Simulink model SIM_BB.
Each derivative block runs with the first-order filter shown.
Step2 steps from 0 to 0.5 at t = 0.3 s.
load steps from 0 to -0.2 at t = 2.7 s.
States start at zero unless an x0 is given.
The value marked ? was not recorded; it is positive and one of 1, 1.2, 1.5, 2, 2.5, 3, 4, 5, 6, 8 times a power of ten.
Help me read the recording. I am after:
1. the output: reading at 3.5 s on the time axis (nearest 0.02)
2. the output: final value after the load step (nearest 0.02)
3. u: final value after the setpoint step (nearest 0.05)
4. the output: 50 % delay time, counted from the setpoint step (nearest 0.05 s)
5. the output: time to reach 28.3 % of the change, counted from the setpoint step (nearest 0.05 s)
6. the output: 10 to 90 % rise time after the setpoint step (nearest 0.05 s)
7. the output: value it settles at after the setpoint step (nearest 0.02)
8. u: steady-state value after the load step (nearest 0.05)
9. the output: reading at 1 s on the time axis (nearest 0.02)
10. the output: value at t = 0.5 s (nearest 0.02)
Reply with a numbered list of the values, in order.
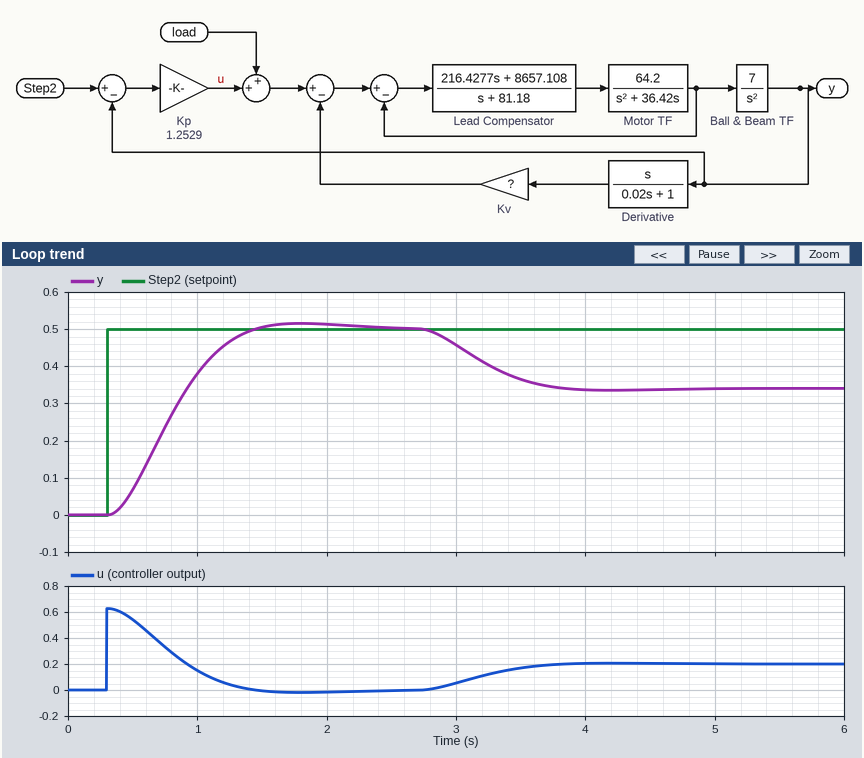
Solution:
1. 0.36
2. 0.34
3. 0.00
4. 0.45 s
5. 0.30 s
6. 0.70 s
7. 0.50
8. 0.20
9. 0.38
10. 0.06
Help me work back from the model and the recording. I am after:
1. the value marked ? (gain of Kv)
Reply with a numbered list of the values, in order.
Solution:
1. 0.6
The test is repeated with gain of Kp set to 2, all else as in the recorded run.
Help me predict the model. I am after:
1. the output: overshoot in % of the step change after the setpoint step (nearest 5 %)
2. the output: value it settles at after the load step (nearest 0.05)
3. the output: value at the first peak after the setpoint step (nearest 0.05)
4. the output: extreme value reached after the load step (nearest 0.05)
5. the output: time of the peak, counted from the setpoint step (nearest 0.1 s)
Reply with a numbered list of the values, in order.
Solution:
1. 10 %
2. 0.40
3. 0.55
4. 0.40
5. 1.0 s
